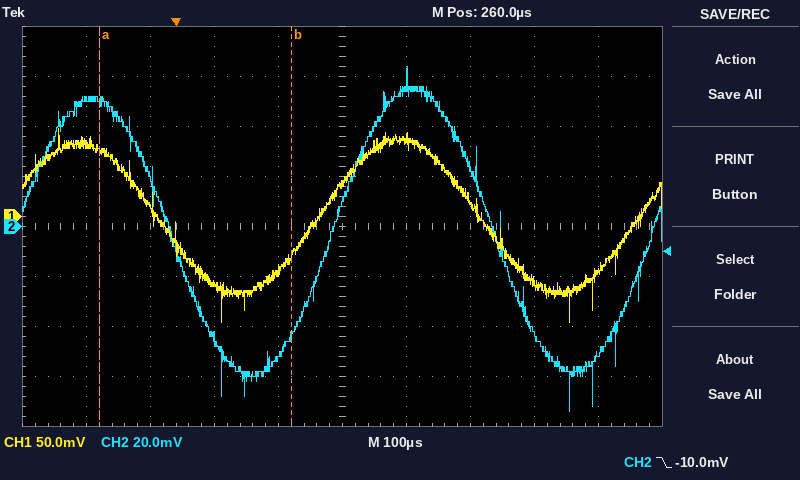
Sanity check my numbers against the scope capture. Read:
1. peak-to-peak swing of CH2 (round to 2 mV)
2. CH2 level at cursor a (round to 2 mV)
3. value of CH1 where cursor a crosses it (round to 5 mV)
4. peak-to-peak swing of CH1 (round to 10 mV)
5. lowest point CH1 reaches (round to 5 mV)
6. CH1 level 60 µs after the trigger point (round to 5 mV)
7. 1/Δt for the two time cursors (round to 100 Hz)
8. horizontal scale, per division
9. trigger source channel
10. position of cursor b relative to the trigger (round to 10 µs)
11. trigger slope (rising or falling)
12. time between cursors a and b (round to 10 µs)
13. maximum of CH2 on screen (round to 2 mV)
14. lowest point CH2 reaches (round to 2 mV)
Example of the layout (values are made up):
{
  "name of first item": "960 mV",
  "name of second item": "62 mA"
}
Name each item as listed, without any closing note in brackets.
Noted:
{
  "peak-to-peak swing of CH2": "138 mV",
  "CH2 level at cursor a": "50 mV",
  "value of CH1 where cursor a crosses it": "65 mV",
  "peak-to-peak swing of CH1": "190 mV",
  "lowest point CH1 reaches": "-105 mV",
  "CH1 level 60 µs after the trigger point": "-70 mV",
  "1/Δt for the two time cursors": "3.3 kHz",
  "horizontal scale, per division": "100 µs",
  "trigger source channel": "CH2",
  "position of cursor b relative to the trigger": "+180 µs",
  "trigger slope": "falling",
  "time between cursors a and b": "300 µs",
  "maximum of CH2 on screen": "64 mV",
  "lowest point CH2 reaches": "-74 mV"
}
